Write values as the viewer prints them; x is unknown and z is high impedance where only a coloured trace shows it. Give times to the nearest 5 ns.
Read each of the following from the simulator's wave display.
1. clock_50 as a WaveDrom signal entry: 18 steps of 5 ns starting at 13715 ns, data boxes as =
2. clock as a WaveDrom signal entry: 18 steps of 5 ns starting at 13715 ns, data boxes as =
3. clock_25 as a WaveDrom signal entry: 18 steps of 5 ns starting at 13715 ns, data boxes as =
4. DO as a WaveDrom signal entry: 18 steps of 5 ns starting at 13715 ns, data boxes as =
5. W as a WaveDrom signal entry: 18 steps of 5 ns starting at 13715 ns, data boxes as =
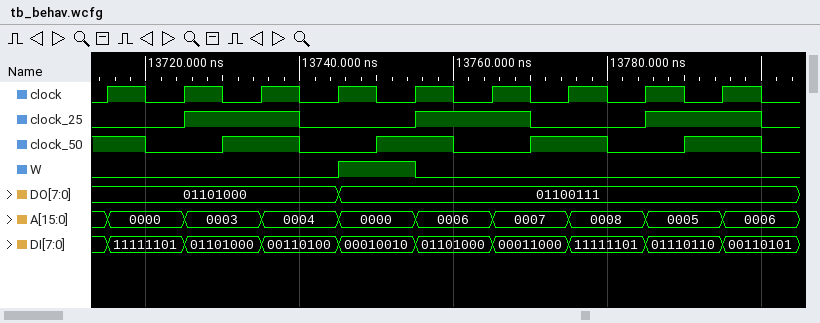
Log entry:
{name: 'clock_50', wave: '10.1.0.1.0.1.0.1.0'}
{name: 'clock', wave: '101010101010101010'}
{name: 'clock_25', wave: '0.1..0..1..0..1..0'}
{name: 'DO', wave: '=.....=...........', data: '01101000 01100111'}
{name: 'W', wave: '0.....1.0.........'}
